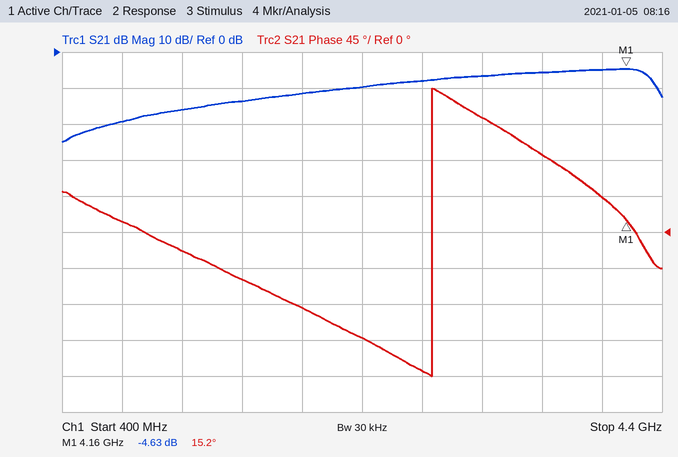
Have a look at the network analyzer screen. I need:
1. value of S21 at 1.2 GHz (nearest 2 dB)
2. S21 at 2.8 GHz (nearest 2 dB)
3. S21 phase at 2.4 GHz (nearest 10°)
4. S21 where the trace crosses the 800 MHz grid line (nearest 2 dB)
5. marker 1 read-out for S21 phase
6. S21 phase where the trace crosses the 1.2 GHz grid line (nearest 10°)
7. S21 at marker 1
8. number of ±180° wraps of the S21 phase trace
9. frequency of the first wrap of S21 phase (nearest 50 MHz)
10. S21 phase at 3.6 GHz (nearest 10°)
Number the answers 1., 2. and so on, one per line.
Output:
1. -16 dB
2. -8 dB
3. -130°
4. -20 dB
5. 15.2°
6. -20°
7. -4.63 dB
8. 1
9. 2.85 GHz
10. 100°
